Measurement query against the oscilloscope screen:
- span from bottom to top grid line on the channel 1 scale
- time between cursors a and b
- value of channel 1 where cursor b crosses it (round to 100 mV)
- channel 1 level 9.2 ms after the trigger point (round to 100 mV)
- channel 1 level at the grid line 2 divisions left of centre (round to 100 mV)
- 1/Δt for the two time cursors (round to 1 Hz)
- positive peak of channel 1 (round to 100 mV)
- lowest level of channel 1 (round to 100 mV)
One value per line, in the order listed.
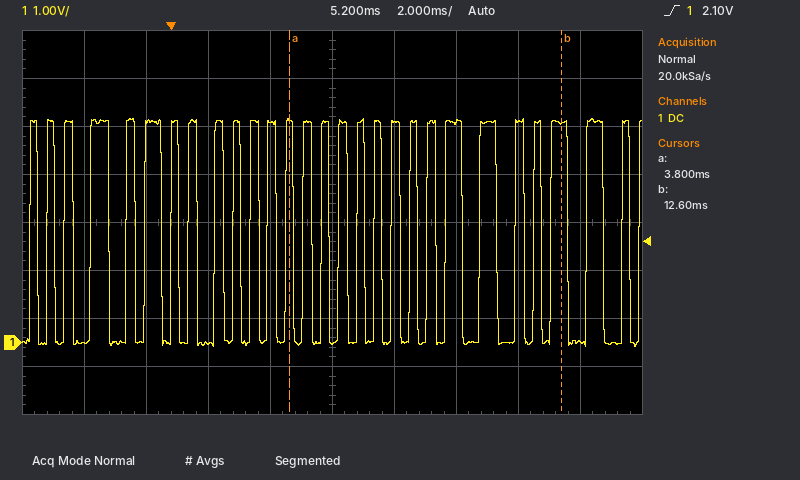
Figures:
8 V
8.8 ms
4.6 V
4.6 V
0.0 V
114 Hz
4.7 V
-100 mV
